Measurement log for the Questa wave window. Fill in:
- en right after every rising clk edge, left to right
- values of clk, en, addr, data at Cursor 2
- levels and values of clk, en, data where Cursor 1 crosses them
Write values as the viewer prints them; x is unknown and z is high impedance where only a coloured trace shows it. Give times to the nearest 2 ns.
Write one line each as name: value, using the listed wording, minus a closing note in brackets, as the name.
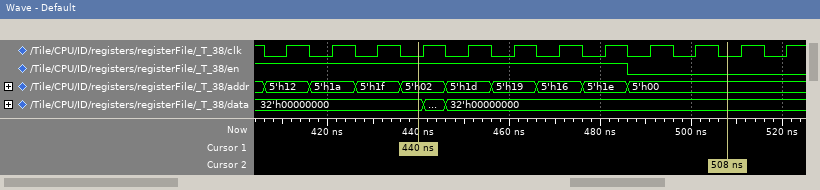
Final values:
en right after every rising clk edge, left to right: 1 1 1 1 1 1 1 1 0 0 0 0
values of clk, en, addr, data at Cursor 2: clk=0, en=0, addr=5'h00, data=32'h00000000
levels and values of clk, en, data where Cursor 1 crosses them: clk=0, en=1, data=32'h00000000
